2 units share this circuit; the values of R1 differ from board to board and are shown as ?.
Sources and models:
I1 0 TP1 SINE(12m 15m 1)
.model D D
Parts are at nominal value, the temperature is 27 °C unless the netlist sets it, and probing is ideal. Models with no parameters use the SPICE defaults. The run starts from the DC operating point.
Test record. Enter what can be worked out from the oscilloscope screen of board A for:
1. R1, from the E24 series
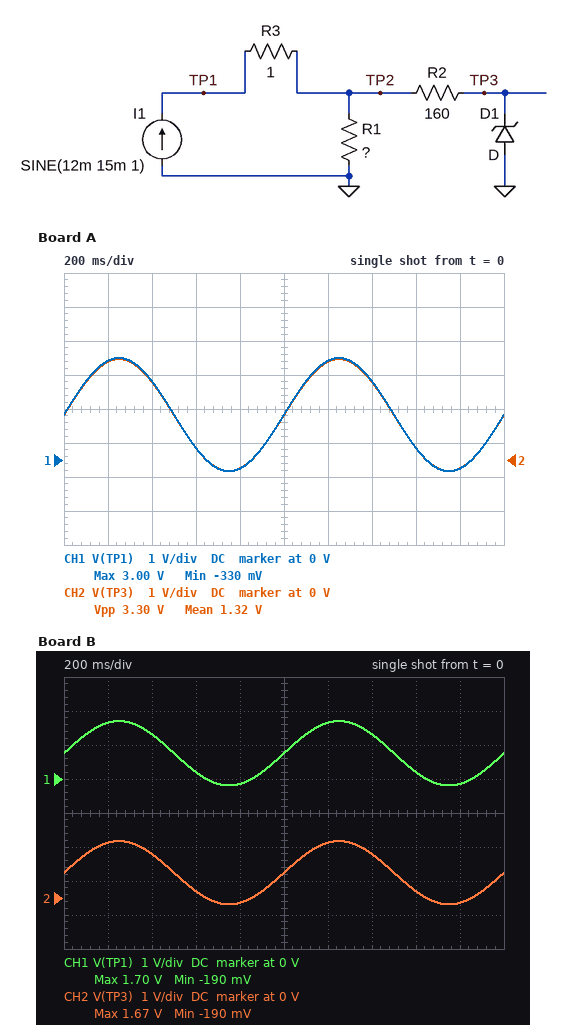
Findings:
110 Ω
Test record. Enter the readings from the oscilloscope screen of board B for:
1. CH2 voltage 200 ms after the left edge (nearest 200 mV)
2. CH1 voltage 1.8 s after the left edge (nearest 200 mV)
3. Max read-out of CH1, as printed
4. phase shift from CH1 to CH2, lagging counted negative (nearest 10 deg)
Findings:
1.6 V
-200 mV
1.70 V
0 deg
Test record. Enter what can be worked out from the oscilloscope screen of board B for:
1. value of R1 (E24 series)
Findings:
62 Ω
